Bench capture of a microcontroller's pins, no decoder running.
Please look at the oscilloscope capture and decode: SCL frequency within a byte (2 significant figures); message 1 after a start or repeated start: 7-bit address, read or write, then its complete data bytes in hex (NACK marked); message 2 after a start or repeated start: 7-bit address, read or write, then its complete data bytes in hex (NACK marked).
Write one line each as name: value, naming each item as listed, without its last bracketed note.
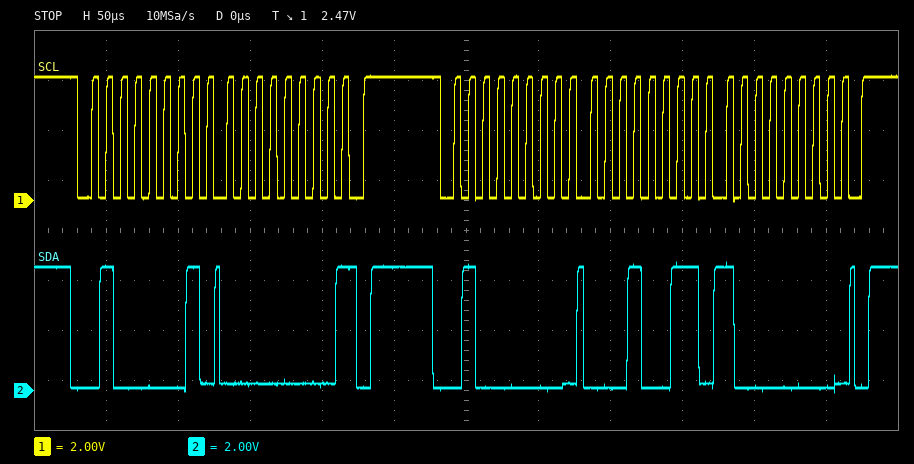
SCL frequency within a byte: 100 kHz
message 1 after a start or repeated start: 7-bit address, read or write, then its complete data bytes in hex: 0x20 read: 00 NACK
message 2 after a start or repeated start: 7-bit address, read or write, then its complete data bytes in hex: 0x20 write: 13 80
